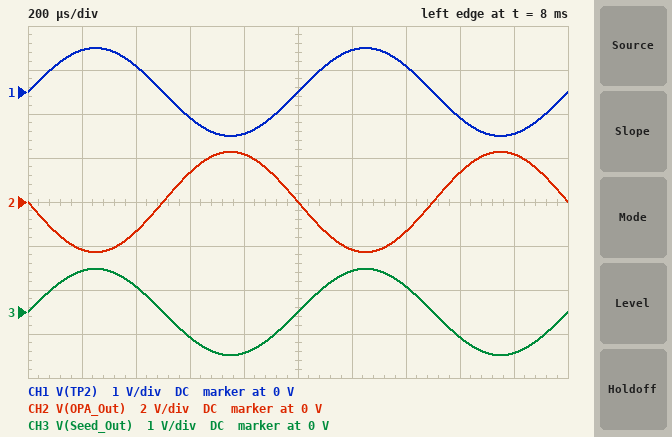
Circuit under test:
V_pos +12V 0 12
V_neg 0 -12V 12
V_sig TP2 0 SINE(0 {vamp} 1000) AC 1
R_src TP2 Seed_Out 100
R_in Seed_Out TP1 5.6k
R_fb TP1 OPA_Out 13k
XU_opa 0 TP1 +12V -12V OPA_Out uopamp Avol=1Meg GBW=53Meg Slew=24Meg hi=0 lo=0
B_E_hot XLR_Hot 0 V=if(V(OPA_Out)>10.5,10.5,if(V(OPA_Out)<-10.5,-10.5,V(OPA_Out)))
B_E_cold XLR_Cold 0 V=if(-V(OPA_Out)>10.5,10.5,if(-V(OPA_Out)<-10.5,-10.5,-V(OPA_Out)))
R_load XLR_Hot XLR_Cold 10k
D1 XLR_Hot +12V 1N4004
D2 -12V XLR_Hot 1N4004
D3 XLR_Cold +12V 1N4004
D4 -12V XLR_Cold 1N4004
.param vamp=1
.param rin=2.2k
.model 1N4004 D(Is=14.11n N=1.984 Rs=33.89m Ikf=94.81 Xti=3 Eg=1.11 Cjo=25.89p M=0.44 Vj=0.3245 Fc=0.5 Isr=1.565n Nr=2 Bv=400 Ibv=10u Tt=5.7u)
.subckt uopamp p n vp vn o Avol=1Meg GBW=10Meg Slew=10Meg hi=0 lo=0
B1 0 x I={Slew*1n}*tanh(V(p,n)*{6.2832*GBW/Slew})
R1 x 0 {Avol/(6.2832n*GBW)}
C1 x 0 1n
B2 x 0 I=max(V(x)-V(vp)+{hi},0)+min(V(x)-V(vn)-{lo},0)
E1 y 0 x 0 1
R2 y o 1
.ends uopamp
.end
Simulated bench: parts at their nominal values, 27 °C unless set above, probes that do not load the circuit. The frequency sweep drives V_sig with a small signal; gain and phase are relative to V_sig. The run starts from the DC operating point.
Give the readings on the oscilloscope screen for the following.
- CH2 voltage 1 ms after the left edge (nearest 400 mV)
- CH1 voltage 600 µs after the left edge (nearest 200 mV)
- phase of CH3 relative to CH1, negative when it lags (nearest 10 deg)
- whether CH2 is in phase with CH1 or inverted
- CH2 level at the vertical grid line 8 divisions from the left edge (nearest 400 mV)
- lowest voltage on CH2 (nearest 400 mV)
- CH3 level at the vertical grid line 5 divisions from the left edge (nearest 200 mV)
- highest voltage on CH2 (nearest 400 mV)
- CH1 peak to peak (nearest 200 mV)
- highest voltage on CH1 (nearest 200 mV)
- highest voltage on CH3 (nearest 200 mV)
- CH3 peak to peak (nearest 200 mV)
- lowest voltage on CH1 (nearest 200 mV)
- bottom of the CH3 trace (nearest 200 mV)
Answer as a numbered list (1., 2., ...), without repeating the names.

1. 0 V
2. -600 mV
3. 0 deg
4. inverted
5. 1.2 V
6. -2.4 V
7. 0 V
8. 2.4 V
9. 2.0 V
10. 1.0 V
11. 1.0 V
12. 2.0 V
13. -1.0 V
14. -1.0 V
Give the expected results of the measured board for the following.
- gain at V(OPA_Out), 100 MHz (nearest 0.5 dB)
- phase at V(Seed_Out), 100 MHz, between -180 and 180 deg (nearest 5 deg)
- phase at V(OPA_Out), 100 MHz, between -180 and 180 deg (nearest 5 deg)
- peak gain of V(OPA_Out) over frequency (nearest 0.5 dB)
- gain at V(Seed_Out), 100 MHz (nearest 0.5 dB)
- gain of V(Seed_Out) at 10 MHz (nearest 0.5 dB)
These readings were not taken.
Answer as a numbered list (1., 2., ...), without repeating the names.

1. -9.0 dB
2. 0 deg
3. 100 deg
4. 7.0 dB
5. 0 dB
6. 0 dB
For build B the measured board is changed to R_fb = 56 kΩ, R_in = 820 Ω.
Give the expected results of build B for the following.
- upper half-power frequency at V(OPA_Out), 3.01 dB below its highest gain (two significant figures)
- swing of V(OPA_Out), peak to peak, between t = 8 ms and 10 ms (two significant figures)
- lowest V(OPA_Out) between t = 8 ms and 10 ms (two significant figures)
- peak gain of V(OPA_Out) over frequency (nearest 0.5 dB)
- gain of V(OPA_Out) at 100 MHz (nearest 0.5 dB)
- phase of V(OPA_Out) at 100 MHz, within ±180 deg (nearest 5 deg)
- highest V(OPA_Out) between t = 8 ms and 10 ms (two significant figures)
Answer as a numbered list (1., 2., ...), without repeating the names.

1. 860 kHz
2. 24 V
3. -12 V
4. 35.5 dB
5. -5.5 dB
6. 90 deg
7. 12 V
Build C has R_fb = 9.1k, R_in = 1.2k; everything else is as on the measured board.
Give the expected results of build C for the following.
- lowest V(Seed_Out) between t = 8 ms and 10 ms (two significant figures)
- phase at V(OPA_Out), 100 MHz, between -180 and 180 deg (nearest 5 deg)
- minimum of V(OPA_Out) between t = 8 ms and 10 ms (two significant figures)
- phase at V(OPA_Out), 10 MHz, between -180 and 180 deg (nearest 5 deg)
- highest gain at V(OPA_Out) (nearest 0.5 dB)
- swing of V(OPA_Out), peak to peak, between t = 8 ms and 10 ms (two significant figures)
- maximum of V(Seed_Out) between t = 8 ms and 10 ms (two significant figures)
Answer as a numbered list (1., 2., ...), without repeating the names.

1. -920 mV
2. 95 deg
3. -7.0 V
4. 125 deg
5. 17.0 dB
6. 14 V
7. 920 mV
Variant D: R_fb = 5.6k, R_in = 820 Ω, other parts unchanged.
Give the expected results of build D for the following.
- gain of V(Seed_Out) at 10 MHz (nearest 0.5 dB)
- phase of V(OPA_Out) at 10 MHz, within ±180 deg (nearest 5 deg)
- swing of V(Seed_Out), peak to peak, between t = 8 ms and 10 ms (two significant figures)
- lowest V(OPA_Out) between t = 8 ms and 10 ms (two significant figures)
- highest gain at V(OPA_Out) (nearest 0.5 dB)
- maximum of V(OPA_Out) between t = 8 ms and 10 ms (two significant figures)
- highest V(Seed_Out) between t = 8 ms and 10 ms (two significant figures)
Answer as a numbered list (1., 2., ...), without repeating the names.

1. -0.5 dB
2. 125 deg
3. 1.8 V
4. -6.1 V
5. 15.5 dB
6. 6.1 V
7. 890 mV
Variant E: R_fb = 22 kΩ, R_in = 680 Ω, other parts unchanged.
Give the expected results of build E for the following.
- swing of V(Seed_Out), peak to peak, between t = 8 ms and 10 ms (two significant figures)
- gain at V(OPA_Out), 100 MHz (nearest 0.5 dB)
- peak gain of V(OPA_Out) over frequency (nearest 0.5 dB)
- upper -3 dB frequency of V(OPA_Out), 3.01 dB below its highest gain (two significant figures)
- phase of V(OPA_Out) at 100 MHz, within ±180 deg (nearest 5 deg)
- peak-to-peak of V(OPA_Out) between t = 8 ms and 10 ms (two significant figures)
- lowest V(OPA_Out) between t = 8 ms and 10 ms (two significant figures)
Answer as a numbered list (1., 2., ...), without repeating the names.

1. 1.9 V
2. -6.0 dB
3. 29.0 dB
4. 1.8 MHz
5. 90 deg
6. 24 V
7. -12 V
